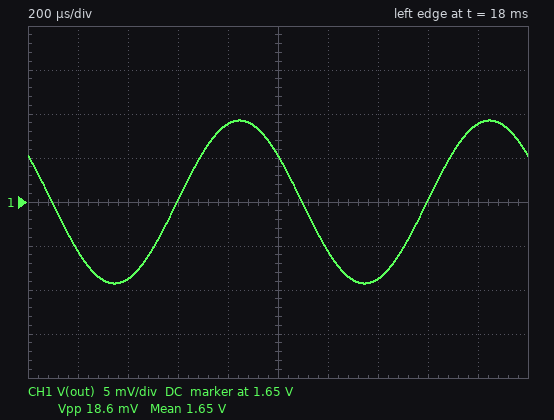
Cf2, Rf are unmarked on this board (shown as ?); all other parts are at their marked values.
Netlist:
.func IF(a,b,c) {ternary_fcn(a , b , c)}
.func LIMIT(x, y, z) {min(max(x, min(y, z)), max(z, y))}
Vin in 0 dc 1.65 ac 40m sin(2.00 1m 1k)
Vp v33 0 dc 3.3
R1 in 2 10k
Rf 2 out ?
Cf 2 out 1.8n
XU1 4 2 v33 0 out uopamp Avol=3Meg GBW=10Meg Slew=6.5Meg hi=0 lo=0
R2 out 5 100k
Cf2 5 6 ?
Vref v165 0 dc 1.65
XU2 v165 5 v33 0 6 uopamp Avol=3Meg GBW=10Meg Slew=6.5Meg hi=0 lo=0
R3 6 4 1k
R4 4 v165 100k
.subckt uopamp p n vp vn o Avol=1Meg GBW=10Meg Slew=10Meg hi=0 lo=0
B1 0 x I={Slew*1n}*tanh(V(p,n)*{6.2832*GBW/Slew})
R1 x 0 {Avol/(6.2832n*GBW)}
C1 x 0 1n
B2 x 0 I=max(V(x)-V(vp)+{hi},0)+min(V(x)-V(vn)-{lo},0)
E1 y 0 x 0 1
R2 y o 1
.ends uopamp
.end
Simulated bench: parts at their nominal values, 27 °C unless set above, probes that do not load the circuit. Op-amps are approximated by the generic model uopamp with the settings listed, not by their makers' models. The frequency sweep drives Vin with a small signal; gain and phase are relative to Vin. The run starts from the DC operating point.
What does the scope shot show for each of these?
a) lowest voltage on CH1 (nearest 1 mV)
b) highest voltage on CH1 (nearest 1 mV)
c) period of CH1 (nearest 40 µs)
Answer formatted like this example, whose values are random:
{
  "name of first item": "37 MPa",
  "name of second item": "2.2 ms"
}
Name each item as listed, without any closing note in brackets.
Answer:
{
  "lowest voltage on CH1": "1.641 V",
  "highest voltage on CH1": "1.659 V",
  "period of CH1": "1.00 ms"
}
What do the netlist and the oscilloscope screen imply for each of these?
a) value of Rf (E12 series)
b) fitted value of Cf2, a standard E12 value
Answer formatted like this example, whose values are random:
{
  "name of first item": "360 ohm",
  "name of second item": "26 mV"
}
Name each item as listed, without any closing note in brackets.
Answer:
{
  "value of Rf": "120 kΩ",
  "fitted value of Cf2, a standard E12 value": "33 nF"
}
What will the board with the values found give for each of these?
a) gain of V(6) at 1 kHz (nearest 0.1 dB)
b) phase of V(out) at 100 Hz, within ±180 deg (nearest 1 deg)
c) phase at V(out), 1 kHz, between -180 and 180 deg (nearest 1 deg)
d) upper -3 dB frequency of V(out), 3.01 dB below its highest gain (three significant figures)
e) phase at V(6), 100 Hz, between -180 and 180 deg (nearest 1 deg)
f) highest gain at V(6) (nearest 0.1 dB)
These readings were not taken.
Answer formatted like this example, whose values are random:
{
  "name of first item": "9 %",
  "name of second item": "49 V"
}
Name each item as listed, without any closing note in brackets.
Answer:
{
  "gain of V(6) at 1 kHz": "-7.0 dB",
  "phase of V(out) at 100 Hz, within ±180 deg": "-100 deg",
  "phase at V(out), 1 kHz, between -180 and 180 deg": "145 deg",
  "upper -3 dB frequency of V(out), 3.01 dB below its highest gain": "1.17 kHz",
  "phase at V(6), 100 Hz, between -180 and 180 deg": "-10 deg",
  "highest gain at V(6)": "-0.1 dB"
}
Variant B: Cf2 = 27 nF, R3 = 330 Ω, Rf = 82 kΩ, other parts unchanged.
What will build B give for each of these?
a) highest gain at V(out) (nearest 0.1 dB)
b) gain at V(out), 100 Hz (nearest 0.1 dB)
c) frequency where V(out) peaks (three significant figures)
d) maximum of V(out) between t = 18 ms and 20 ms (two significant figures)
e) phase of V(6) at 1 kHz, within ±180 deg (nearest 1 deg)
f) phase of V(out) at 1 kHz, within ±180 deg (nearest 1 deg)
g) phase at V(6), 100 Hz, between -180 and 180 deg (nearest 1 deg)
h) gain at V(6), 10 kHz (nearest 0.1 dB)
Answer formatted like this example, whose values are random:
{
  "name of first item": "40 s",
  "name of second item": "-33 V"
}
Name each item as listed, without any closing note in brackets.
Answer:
{
  "highest gain at V(out)": "17.8 dB",
  "gain at V(out), 100 Hz": "3.6 dB",
  "frequency where V(out) peaks": "763 Hz",
  "maximum of V(out) between t = 18 ms and 20 ms": "1.7 V",
  "phase of V(6) at 1 kHz, within ±180 deg": "-110 deg",
  "phase of V(out) at 1 kHz, within ±180 deg": "160 deg",
  "phase at V(6), 100 Hz, between -180 and 180 deg": "-11 deg",
  "gain at V(6), 10 kHz": "-45.7 dB"
}
